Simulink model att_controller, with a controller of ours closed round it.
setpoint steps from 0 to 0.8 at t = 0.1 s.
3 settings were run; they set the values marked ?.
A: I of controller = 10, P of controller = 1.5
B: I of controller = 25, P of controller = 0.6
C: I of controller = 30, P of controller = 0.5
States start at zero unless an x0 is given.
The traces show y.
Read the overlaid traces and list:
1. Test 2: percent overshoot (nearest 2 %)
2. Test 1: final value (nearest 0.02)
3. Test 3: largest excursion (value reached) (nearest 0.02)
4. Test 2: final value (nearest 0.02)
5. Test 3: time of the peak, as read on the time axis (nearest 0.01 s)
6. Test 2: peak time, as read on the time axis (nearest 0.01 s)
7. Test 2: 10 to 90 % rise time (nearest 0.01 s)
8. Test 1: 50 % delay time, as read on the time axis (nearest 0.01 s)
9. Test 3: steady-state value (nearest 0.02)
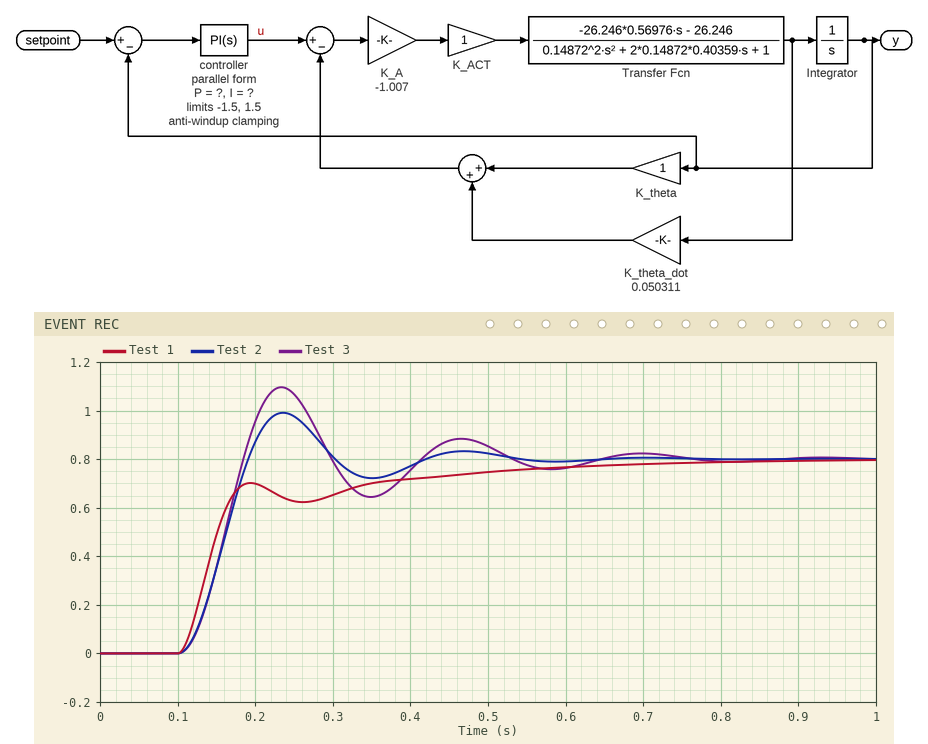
24 %
0.80
1.10
0.80
0.23 s
0.24 s
0.06 s
0.14 s
0.80
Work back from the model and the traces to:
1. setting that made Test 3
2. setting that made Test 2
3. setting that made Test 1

C
B
A
